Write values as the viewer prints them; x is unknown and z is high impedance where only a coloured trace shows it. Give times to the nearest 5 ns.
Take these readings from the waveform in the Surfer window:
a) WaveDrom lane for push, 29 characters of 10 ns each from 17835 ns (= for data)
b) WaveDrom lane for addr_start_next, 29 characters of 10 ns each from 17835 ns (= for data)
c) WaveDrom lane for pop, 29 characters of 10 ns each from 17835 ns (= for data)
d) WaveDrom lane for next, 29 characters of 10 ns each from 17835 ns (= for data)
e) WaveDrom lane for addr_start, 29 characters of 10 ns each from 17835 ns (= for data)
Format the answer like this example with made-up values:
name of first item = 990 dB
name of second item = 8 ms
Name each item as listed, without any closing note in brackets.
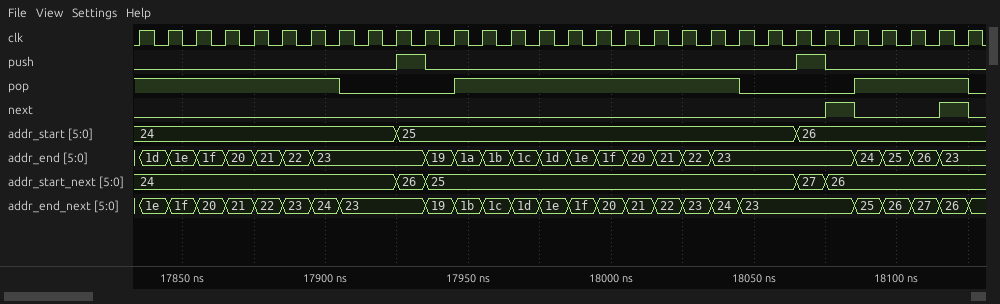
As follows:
WaveDrom lane for push, 29 characters of 10 ns each from 17835 ns = {name: 'push', wave: '0........10............10....'}
WaveDrom lane for addr_start_next, 29 characters of 10 ns each from 17835 ns = {name: 'addr_start_next', wave: '=........==............==....', data: '24 26 25 27 26'}
WaveDrom lane for pop, 29 characters of 10 ns each from 17835 ns = {name: 'pop', wave: '1......0...1.........0...1...'}
WaveDrom lane for next, 29 characters of 10 ns each from 17835 ns = {name: 'next', wave: '0.......................10..1'}
WaveDrom lane for addr_start, 29 characters of 10 ns each from 17835 ns = {name: 'addr_start', wave: '=........=.............=.....', data: '24 25 26'}
